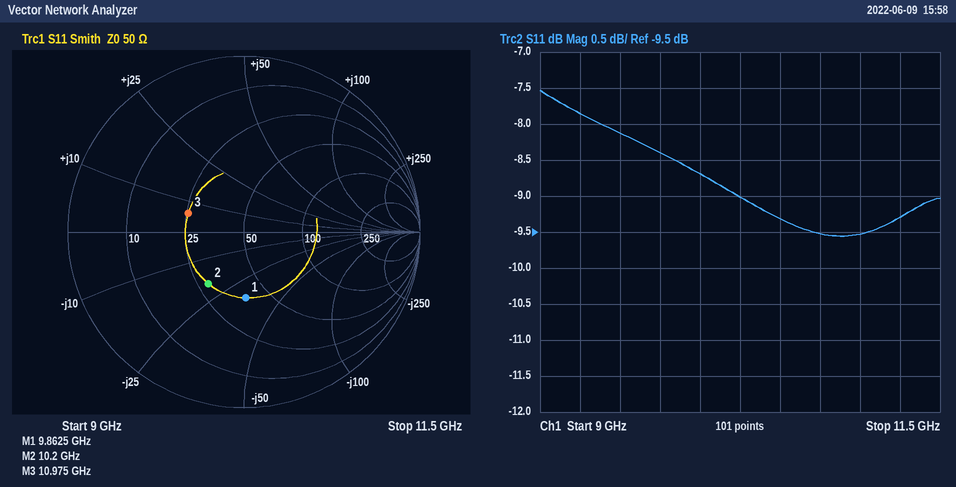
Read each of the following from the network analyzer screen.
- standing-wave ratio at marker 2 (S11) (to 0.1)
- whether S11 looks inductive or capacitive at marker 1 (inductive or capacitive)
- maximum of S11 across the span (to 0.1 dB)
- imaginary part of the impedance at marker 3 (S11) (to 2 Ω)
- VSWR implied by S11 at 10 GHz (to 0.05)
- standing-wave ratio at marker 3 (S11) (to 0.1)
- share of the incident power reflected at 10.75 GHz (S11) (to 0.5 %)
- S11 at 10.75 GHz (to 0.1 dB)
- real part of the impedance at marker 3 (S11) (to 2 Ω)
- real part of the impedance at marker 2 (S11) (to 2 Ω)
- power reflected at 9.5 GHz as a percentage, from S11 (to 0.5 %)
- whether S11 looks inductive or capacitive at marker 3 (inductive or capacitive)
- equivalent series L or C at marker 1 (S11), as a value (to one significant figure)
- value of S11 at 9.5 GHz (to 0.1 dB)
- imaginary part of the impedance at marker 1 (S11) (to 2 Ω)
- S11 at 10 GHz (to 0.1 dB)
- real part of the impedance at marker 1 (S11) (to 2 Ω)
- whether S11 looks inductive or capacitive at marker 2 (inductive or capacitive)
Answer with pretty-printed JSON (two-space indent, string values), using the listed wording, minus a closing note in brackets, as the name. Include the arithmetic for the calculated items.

{
  "standing-wave ratio at marker 2 (S11)": "2.1",
  "whether S11 looks inductive or capacitive at marker 1": "capacitive",
  "maximum of S11 across the span": "-7.5 dB",
  "imaginary part of the impedance at marker 3 (S11)": "+6 Ω",
  "VSWR implied by S11 at 10 GHz": "|Γ| = 10^(-8.7/20) = 0.3673; VSWR = (1 + 0.3673)/(1 − 0.3673) ≈ 2.16, so 2.15 to the nearest 0.05",
  "standing-wave ratio at marker 3 (S11)": "2.0",
  "share of the incident power reflected at 10.75 GHz (S11)": "10^(-9.5/10) ≈ 11.2 %, so 11.0 % to the nearest 0.5 %",
  "S11 at 10.75 GHz": "-9.5 dB",
  "real part of the impedance at marker 3 (S11)": "26 Ω",
  "real part of the impedance at marker 2 (S11)": "28 Ω",
  "power reflected at 9.5 GHz as a percentage, from S11": "10^(-8.1/10) ≈ 15.5 %",
  "whether S11 looks inductive or capacitive at marker 3": "inductive",
  "equivalent series L or C at marker 1 (S11), as a value": "C = 1/(2π × 9.8625 GHz × 34 Ω) ≈ 475 fF, so 500 fF to one significant figure",
  "value of S11 at 9.5 GHz": "-8.1 dB",
  "imaginary part of the impedance at marker 1 (S11)": "-34 Ω",
  "S11 at 10 GHz": "-8.7 dB",
  "real part of the impedance at marker 1 (S11)": "38 Ω",
  "whether S11 looks inductive or capacitive at marker 2": "capacitive"
}
